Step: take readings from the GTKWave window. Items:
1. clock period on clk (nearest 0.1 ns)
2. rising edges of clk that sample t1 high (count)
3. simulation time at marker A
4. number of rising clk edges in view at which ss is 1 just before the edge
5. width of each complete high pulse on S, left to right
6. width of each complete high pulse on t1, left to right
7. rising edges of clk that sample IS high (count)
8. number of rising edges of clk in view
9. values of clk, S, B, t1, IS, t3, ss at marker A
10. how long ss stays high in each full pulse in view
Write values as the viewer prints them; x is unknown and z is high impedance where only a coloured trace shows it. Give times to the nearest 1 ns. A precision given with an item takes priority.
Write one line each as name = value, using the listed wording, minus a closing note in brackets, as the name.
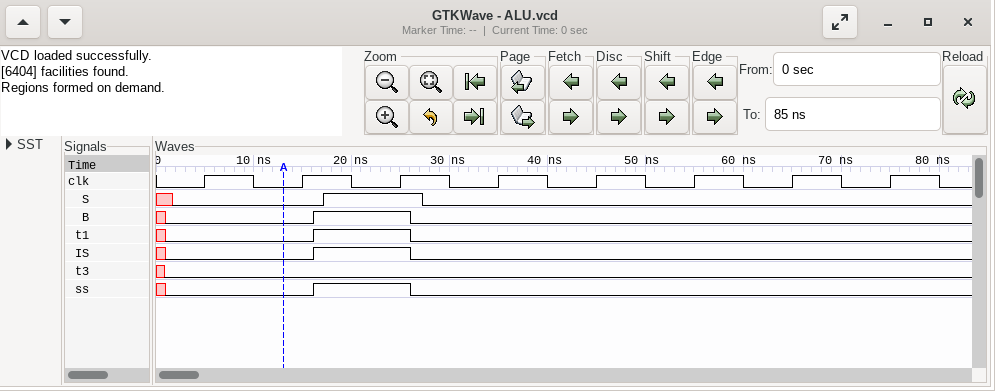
clock period on clk = 10 ns
rising edges of clk that sample t1 high = 1
simulation time at marker A = 13 ns
number of rising clk edges in view at which ss is 1 just before the edge = 1
width of each complete high pulse on S, left to right = 10 ns
width of each complete high pulse on t1, left to right = 10 ns
rising edges of clk that sample IS high = 1
number of rising edges of clk in view = 8
values of clk, S, B, t1, IS, t3, ss at marker A = clk=0, S=0, B=0, t1=0, IS=0, t3=0, ss=0
how long ss stays high in each full pulse in view = 10 ns
